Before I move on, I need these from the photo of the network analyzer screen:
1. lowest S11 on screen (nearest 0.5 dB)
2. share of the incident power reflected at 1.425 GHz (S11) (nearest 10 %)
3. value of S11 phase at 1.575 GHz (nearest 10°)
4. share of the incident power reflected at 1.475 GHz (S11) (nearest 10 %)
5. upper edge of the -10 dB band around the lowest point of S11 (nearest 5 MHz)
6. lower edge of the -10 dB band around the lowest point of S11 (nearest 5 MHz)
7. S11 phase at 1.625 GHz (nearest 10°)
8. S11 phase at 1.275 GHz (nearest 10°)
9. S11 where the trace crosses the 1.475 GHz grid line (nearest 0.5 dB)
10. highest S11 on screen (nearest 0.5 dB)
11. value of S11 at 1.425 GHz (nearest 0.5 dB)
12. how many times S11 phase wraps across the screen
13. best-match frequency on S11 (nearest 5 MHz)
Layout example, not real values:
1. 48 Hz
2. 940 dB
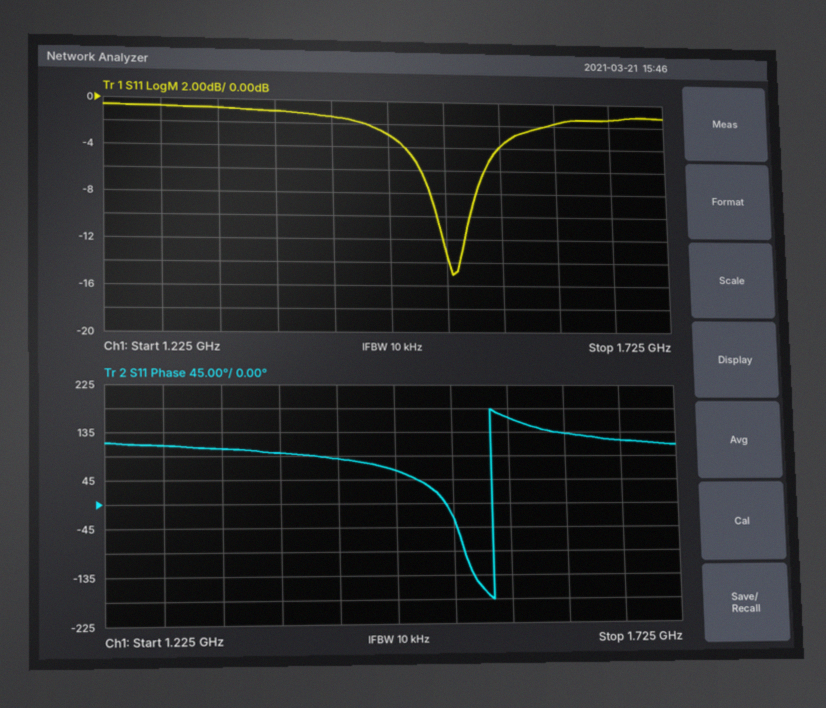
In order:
1. -15.0 dB
2. 70 %
3. 160°
4. 50 %
5. 1.545 GHz
6. 1.515 GHz
7. 130°
8. 110°
9. -3.0 dB
10. -0.5 dB
11. -1.5 dB
12. 1
13. 1.530 GHz
